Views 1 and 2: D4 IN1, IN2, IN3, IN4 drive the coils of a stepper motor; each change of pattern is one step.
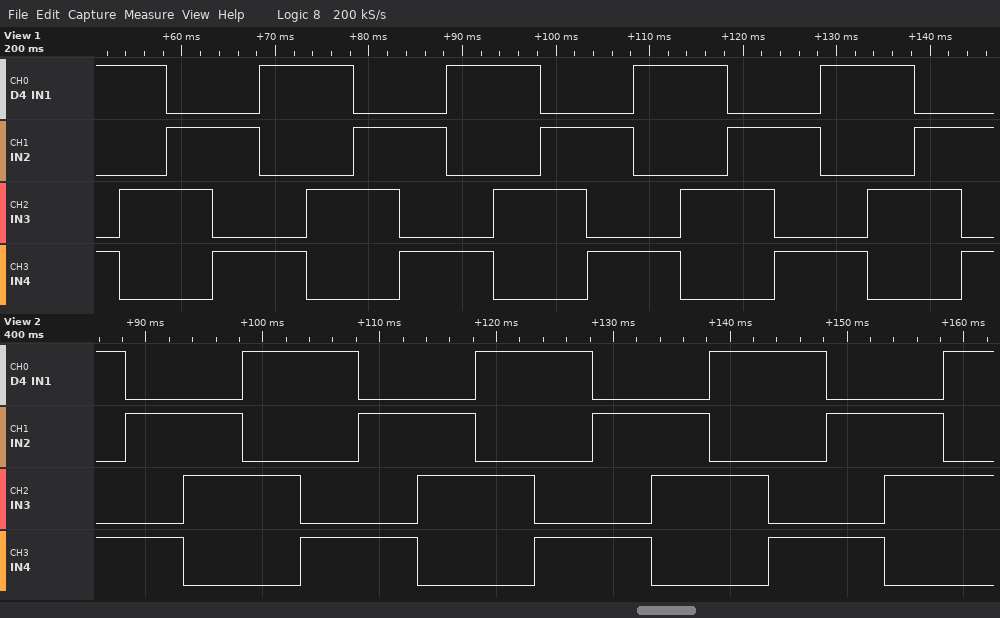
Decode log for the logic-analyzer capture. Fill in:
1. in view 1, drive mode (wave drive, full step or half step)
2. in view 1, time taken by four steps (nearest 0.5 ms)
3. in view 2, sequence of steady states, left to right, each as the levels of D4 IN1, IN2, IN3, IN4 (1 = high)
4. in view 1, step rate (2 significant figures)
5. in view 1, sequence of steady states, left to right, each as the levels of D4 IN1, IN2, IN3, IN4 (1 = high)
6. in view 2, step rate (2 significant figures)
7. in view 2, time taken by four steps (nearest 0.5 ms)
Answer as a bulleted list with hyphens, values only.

- full step
- 20.0 ms
- 1001 0101 0110 1010 1001 0101 0110 1010 1001 0101 0110 1010 1001 0101 0110 1010
- 200 steps/s
- 1001 1010 0110 0101 1001 1010 0110 0101 1001 1010 0110 0101 1001 1010 0110 0101 1001 1010 0110 0101
- 200 steps/s
- 20.0 ms
